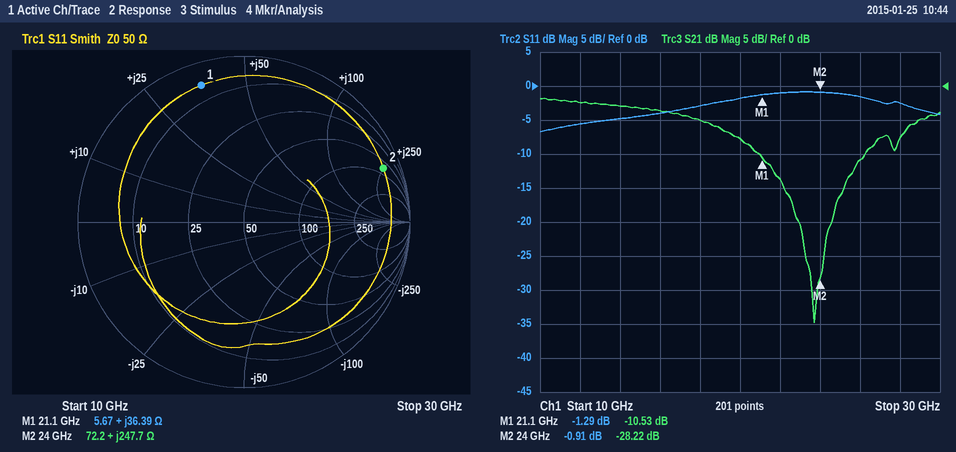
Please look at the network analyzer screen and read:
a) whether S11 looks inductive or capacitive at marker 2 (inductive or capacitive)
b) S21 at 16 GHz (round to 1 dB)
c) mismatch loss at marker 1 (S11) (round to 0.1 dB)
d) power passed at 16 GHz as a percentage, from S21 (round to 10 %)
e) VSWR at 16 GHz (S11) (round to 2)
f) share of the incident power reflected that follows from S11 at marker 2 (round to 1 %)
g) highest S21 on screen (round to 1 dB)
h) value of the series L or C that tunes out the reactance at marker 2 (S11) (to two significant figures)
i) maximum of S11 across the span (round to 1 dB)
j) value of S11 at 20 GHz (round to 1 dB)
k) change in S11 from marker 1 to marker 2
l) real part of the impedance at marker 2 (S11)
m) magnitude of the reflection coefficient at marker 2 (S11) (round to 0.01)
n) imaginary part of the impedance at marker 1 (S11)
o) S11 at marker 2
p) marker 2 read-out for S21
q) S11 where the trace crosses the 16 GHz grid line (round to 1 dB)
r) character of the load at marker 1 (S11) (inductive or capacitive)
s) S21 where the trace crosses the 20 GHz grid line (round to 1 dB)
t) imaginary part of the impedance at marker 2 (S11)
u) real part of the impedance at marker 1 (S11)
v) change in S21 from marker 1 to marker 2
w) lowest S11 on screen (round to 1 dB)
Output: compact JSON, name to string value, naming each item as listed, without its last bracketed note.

{"whether S11 looks inductive or capacitive at marker 2": "inductive", "S21 at 16 GHz": "-4 dB", "mismatch loss at marker 1 (S11)": "5.9 dB", "power passed at 16 GHz as a percentage, from S21": "40 %", "VSWR at 16 GHz (S11)": "4", "share of the incident power reflected that follows from S11 at marker 2": "81 %", "highest S21 on screen": "-2 dB", "value of the series L or C that tunes out the reactance at marker 2 (S11)": "27 fF", "maximum of S11 across the span": "-1 dB", "value of S11 at 20 GHz": "-2 dB", "change in S11 from marker 1 to marker 2": "0.38 dB", "real part of the impedance at marker 2": "72.2 Ω", "magnitude of the reflection coefficient at marker 2 (S11)": "0.90", "imaginary part of the impedance at marker 1": "+36.39 Ω", "S11 at marker 2": "-0.91 dB", "marker 2 read-out for S21": "-28.22 dB", "S11 where the trace crosses the 16 GHz grid line": "-4 dB", "character of the load at marker 1 (S11)": "inductive", "S21 where the trace crosses the 20 GHz grid line": "-8 dB", "imaginary part of the impedance at marker 2": "+247.7 Ω", "real part of the impedance at marker 1": "5.67 Ω", "change in S21 from marker 1 to marker 2": "-17.69 dB", "lowest S11 on screen": "-7 dB"}
